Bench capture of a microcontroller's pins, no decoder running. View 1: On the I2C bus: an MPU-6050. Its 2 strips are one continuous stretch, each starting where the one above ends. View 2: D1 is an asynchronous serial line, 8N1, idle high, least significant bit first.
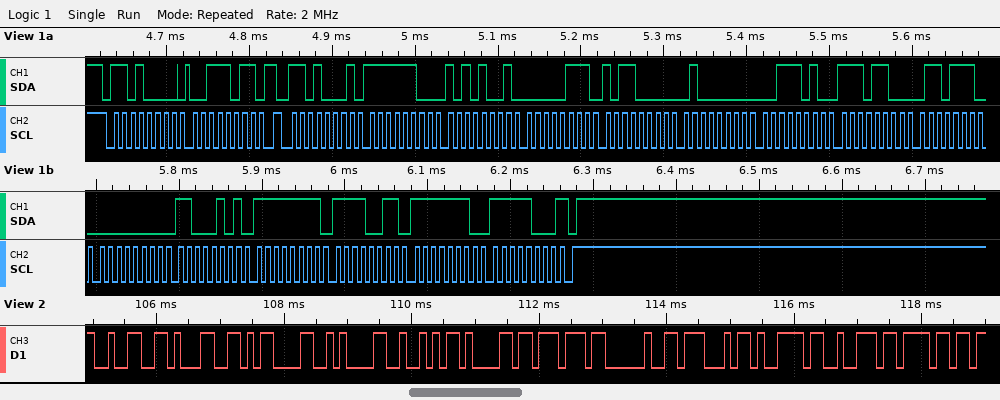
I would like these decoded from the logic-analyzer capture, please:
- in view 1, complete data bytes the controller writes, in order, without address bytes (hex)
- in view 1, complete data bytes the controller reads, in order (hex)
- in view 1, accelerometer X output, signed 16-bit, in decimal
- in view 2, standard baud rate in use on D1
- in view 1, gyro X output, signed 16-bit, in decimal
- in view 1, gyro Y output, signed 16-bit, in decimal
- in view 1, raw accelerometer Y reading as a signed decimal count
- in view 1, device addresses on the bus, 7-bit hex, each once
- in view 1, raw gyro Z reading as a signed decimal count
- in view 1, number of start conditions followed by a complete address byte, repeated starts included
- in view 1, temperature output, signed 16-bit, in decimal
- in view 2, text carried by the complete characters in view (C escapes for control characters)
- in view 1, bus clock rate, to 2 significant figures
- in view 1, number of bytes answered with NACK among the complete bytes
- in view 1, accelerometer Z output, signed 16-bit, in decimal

3B
FC A9 07 B0 40 3A EC 6E 00 C5 FF F3 FE F8
-855
9600 baud
197
-13
1968
0x68
-264
2
-5010
"21\r\nRaw Gyro"
100 kHz
1
16442
